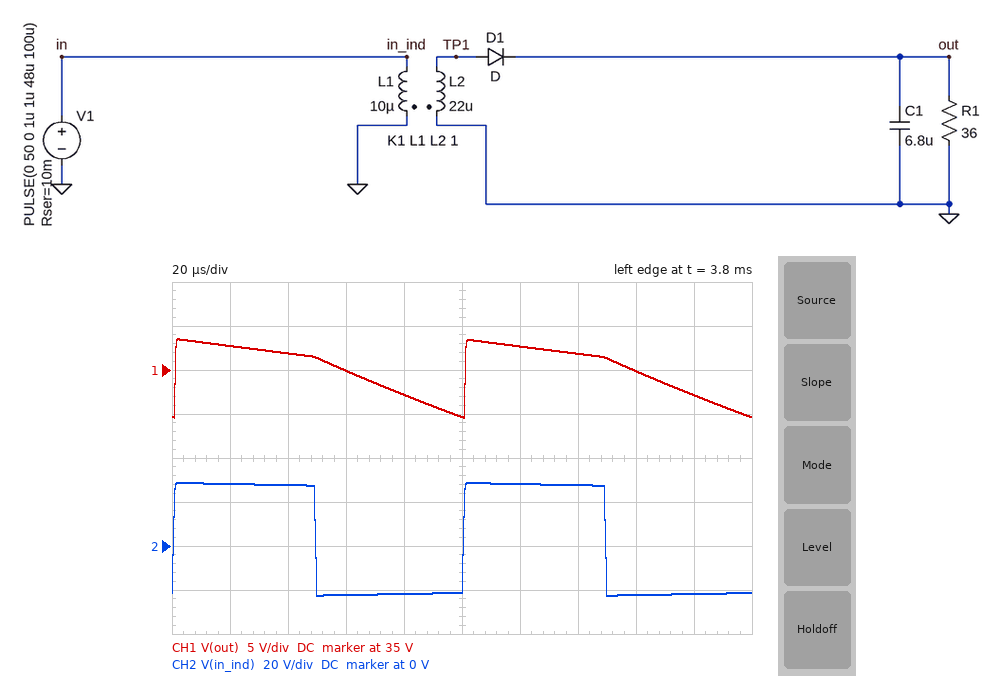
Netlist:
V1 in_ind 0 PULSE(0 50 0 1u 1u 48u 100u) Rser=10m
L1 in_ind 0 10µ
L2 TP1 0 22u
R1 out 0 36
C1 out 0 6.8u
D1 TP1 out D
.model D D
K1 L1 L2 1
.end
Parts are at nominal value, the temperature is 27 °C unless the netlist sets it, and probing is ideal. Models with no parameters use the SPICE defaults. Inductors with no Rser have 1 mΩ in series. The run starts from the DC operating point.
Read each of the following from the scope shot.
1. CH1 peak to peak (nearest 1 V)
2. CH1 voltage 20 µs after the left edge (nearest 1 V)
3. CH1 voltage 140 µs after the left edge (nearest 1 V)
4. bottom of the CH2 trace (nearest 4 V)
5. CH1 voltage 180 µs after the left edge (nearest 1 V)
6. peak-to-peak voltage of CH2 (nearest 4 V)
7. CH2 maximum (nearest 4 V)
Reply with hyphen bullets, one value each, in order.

- 9 V
- 38 V
- 37 V
- -24 V
- 32 V
- 52 V
- 28 V
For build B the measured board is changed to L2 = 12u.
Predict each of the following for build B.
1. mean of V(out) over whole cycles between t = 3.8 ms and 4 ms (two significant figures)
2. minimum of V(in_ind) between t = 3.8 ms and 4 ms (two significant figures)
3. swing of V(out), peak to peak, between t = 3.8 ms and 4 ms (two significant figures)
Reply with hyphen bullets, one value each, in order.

- 26 V
- -23 V
- 6.6 V
